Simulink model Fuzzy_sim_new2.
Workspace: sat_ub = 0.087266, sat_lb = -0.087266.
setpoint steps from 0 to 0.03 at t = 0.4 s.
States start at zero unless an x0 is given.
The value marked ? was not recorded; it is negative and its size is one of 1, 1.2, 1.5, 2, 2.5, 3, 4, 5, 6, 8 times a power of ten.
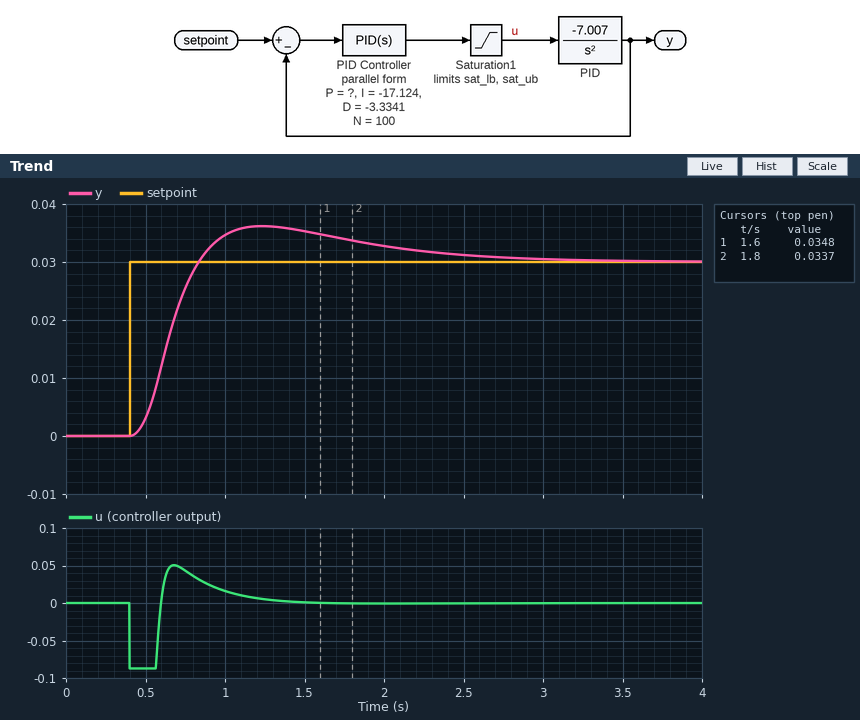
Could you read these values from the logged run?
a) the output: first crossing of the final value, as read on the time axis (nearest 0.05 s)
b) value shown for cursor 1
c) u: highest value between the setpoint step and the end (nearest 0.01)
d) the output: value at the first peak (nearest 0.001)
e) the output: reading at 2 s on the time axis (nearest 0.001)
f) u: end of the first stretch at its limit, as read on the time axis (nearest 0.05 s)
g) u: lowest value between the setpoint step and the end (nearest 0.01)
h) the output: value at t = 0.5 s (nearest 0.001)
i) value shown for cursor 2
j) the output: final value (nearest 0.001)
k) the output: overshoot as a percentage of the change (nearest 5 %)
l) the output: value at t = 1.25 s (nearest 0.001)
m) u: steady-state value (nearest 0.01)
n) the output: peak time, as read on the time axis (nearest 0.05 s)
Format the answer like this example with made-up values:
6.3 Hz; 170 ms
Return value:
0.85 s; 0.0348; 0.05; 0.036; 0.033; 0.55 s; -0.09; 0.003; 0.0337; 0.030; 20 %; 0.036; 0.00; 1.25 s
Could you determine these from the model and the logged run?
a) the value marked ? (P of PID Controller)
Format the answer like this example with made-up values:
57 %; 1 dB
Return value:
-15
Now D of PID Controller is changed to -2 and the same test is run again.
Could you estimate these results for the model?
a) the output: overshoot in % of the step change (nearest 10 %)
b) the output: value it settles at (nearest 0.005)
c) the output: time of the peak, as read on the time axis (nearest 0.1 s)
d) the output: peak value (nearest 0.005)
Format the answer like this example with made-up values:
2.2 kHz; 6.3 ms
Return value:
30 %; 0.030; 0.9 s; 0.040
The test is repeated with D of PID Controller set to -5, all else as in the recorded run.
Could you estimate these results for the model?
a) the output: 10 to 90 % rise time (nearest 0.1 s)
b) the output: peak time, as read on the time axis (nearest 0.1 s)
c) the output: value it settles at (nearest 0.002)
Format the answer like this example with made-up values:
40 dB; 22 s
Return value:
0.4 s; 1.5 s; 0.030
